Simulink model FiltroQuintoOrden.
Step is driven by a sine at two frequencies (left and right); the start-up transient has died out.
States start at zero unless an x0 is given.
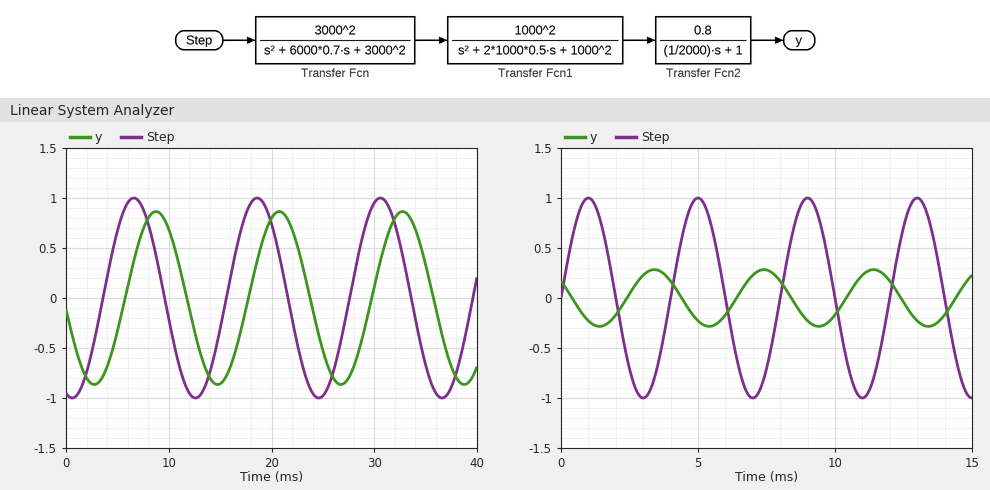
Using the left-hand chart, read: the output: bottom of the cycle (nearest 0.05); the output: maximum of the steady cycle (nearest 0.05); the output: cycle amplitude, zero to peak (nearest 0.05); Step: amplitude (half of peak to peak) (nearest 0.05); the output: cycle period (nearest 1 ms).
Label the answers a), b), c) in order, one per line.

a) -0.85
b) 0.85
c) 0.85
d) 1.00
e) 12 ms
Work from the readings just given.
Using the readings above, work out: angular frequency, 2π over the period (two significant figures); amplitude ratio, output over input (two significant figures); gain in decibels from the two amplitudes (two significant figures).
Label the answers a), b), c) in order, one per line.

a) 0.52 rad/ms
b) 0.85
c) -1.4 dB
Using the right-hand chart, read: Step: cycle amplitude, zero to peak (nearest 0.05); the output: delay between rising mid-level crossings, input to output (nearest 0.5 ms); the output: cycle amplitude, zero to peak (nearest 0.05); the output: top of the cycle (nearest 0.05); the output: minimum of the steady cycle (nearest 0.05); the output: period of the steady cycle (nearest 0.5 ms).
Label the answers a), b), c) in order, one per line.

a) 1.00
b) 2.5 ms
c) 0.30
d) 0.30
e) -0.30
f) 4.0 ms
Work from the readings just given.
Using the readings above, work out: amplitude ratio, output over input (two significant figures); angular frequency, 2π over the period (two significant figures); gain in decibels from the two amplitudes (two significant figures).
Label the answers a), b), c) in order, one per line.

a) 0.30
b) 1.6 rad/ms
c) -10 dB
